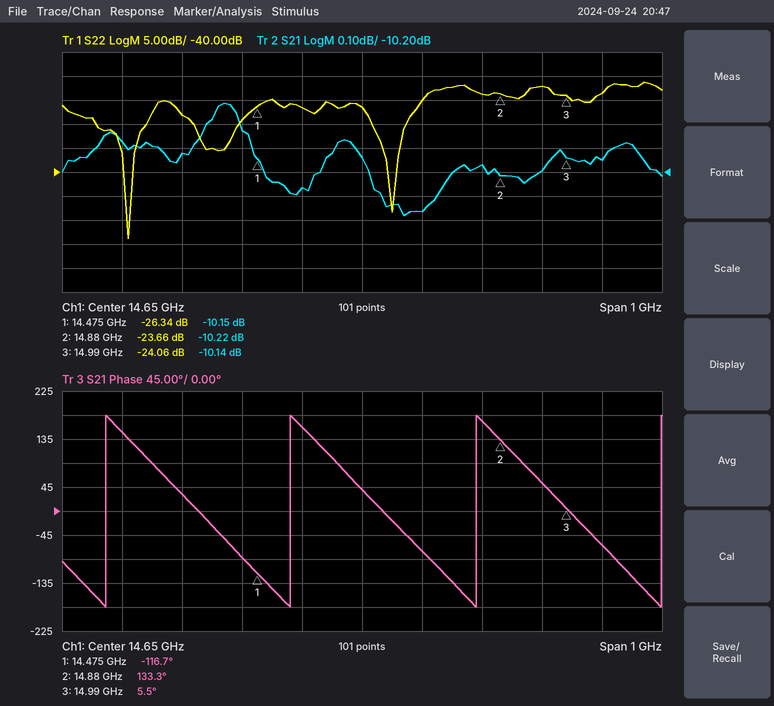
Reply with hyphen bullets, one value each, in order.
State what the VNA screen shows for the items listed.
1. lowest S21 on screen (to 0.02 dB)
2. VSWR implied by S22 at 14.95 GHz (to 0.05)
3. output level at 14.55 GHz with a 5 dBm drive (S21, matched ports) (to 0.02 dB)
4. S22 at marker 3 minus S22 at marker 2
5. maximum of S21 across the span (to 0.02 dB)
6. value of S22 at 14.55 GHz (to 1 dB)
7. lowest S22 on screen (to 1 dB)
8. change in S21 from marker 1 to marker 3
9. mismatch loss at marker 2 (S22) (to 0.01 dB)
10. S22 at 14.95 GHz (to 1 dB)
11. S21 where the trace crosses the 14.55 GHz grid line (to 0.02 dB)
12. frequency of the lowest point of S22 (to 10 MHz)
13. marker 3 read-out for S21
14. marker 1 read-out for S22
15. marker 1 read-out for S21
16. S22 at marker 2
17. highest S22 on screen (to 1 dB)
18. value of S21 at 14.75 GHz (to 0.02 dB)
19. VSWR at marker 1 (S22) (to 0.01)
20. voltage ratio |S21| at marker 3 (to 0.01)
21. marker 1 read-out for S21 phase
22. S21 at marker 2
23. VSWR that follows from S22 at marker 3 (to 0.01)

- -10.38 dB
- 1.15
- -5.26 dBm
- -0.40 dB
- -9.92 dB
- -27 dB
- -54 dB
- 0.01 dB
- 0.02 dB
- -22 dB
- -10.26 dB
- 14.26 GHz
- -10.14 dB
- -26.34 dB
- -10.15 dB
- -23.66 dB
- -21 dB
- -10.36 dB
- 1.10
- 0.31
- -116.7°
- -10.22 dB
- 1.13
